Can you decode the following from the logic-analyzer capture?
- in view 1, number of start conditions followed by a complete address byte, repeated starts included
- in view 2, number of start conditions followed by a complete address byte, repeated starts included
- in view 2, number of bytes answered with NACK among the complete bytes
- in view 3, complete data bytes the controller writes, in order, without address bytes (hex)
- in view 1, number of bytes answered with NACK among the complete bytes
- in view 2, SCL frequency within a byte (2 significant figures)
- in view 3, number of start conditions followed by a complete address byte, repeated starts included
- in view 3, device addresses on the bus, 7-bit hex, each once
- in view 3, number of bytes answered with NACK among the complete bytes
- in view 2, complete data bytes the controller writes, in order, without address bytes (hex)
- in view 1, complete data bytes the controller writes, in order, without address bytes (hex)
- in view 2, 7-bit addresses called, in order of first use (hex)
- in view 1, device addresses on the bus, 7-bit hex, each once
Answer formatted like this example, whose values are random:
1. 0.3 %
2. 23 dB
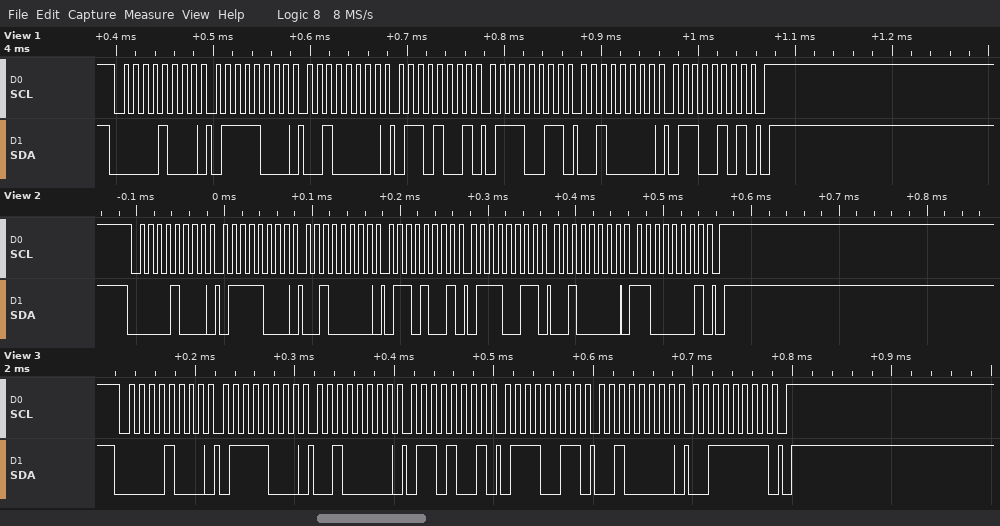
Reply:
1. 1
2. 1
3. 0
4. 78 20 69 73 20 3F
5. 0
6. 100 kHz
7. 1
8. 0x04
9. 0
10. 78 20 69 73 20 C1
11. 78 20 69 73 20 65
12. 0x04
13. 0x04
